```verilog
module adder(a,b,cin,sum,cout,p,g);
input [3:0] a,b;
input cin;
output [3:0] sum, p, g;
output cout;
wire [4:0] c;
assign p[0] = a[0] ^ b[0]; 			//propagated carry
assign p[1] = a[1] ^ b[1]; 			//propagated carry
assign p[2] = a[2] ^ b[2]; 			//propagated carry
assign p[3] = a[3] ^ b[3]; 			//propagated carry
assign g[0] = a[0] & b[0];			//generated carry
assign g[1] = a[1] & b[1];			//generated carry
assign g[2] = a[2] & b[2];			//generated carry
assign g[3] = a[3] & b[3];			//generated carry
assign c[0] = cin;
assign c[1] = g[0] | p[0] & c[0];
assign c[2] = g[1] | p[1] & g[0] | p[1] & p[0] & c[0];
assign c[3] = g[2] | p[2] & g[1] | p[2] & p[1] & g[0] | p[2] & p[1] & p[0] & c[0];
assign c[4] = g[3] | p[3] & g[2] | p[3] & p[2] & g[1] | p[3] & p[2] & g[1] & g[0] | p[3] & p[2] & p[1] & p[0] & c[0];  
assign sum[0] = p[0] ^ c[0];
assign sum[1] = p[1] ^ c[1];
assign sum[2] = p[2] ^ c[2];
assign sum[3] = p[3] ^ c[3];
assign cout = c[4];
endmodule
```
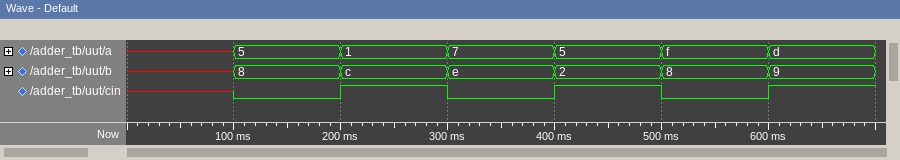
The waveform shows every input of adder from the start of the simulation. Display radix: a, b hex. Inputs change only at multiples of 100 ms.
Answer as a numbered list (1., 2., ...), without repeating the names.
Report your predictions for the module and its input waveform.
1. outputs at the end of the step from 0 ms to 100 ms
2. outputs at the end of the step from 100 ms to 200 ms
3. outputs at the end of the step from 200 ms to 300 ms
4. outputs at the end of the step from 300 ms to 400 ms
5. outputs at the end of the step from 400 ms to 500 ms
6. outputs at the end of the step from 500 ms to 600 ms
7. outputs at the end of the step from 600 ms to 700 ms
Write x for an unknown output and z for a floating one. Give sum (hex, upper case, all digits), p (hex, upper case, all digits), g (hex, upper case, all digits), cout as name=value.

1. sum=x, p=x, g=x, cout=x
2. sum=D, p=D, g=0, cout=0
3. sum=E, p=D, g=0, cout=0
4. sum=5, p=9, g=6, cout=1
5. sum=8, p=7, g=0, cout=0
6. sum=7, p=7, g=8, cout=1
7. sum=7, p=4, g=9, cout=1
